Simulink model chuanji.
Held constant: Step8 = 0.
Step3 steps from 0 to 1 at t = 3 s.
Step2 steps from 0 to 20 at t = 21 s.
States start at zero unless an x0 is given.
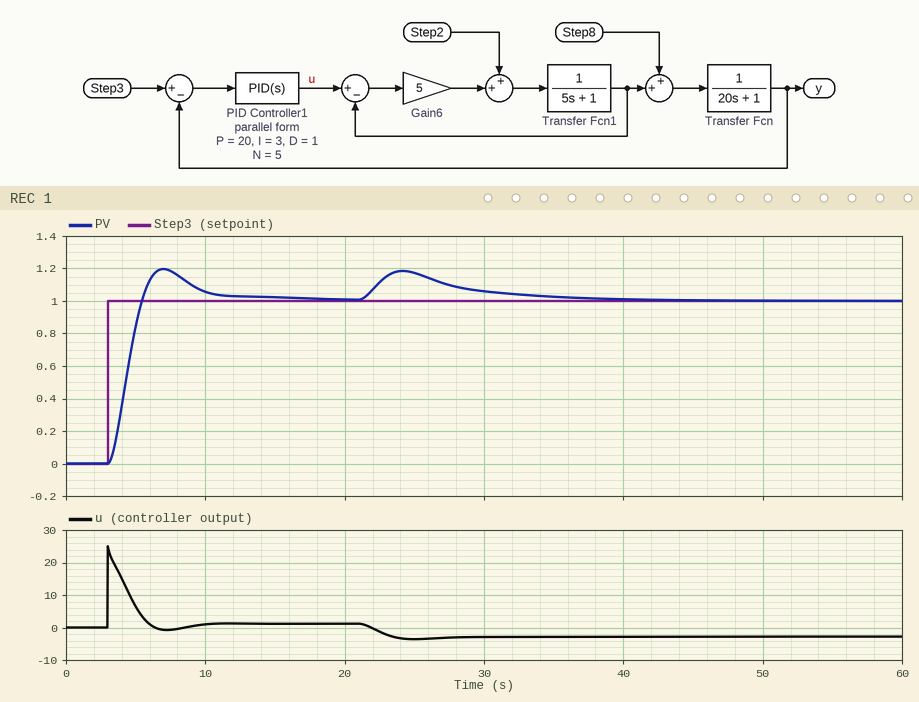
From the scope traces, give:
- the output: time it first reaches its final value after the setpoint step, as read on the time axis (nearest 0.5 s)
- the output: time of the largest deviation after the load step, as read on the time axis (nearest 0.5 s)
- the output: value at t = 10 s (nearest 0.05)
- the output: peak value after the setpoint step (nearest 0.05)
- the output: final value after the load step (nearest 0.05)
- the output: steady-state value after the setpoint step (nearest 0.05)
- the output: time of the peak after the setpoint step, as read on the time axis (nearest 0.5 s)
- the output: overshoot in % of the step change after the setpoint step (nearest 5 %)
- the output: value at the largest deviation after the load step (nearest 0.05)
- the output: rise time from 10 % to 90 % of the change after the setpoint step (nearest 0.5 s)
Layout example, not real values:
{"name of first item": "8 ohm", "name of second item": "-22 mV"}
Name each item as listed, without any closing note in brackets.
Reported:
{"the output: time it first reaches its final value after the setpoint step, as read on the time axis": "5.5 s", "the output: time of the largest deviation after the load step, as read on the time axis": "24.0 s", "the output: value at t = 10 s": "1.05", "the output: peak value after the setpoint step": "1.20", "the output: final value after the load step": "1.00", "the output: steady-state value after the setpoint step": "1.00", "the output: time of the peak after the setpoint step, as read on the time axis": "7.0 s", "the output: overshoot in % of the step change after the setpoint step": "20 %", "the output: value at the largest deviation after the load step": "1.20", "the output: rise time from 10 % to 90 % of the change after the setpoint step": "1.5 s"}
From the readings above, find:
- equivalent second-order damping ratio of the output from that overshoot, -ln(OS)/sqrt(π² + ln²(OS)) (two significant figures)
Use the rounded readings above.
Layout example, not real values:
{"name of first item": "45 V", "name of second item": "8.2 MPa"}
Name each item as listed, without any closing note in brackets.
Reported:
{"equivalent second-order damping ratio of the output from that overshoot, -ln(OS)/sqrt(π² + ln²(OS))": "0.46"}
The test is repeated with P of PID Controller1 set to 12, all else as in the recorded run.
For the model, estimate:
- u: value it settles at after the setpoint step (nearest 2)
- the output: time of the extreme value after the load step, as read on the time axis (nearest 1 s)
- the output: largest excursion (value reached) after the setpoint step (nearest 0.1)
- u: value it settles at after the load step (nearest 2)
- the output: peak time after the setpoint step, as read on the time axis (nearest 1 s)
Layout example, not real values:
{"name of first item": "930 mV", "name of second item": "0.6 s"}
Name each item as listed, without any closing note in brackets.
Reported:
{"u: value it settles at after the setpoint step": "2", "the output: time of the extreme value after the load step, as read on the time axis": "25 s", "the output: largest excursion (value reached) after the setpoint step": "1.3", "u: value it settles at after the load step": "-2", "the output: peak time after the setpoint step, as read on the time axis": "9 s"}
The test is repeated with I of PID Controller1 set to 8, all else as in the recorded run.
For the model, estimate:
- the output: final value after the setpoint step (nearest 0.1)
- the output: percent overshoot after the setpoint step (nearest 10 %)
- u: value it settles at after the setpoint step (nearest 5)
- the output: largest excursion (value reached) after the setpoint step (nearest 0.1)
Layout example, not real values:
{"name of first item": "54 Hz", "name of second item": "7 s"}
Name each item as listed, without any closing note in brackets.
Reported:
{"the output: final value after the setpoint step": "1.0", "the output: percent overshoot after the setpoint step": "40 %", "u: value it settles at after the setpoint step": "0", "the output: largest excursion (value reached) after the setpoint step": "1.4"}
